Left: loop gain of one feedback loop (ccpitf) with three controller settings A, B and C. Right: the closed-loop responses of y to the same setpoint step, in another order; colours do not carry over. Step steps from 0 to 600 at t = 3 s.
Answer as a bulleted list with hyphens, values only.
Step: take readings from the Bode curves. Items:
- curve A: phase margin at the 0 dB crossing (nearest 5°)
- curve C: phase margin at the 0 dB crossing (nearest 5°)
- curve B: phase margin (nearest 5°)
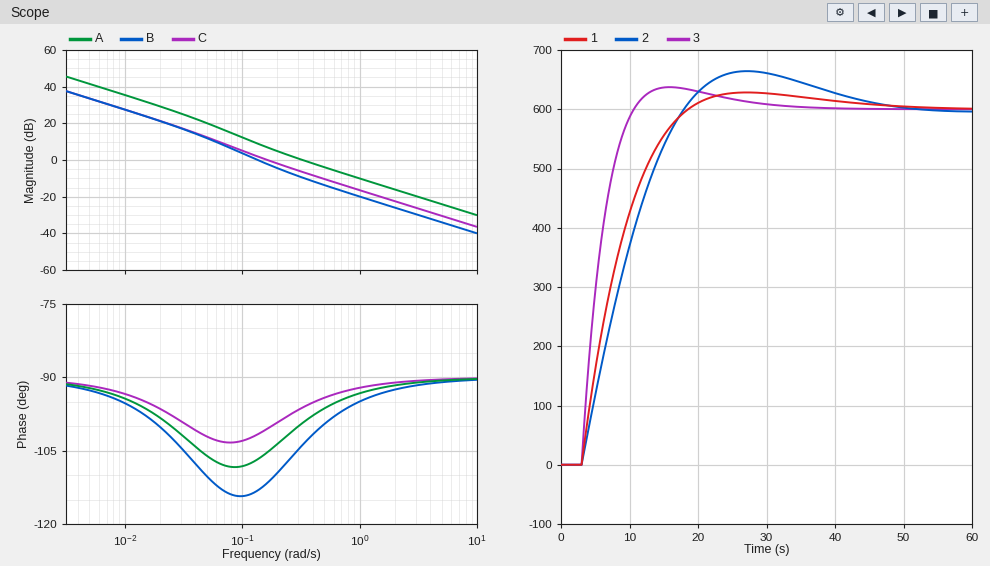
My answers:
- 80°
- 80°
- 65°
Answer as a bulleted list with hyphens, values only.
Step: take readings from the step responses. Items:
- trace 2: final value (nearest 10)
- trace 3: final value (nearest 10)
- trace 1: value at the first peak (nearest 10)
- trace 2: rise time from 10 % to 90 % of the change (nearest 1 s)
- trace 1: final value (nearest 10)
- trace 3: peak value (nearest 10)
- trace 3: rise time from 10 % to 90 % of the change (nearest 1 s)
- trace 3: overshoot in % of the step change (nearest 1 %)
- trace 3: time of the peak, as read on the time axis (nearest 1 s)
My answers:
- 600
- 600
- 630
- 11 s
- 600
- 640
- 5 s
- 6 %
- 16 s
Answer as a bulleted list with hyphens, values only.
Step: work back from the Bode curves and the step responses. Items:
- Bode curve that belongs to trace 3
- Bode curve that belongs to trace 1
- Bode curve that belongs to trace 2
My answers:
- A
- C
- B
